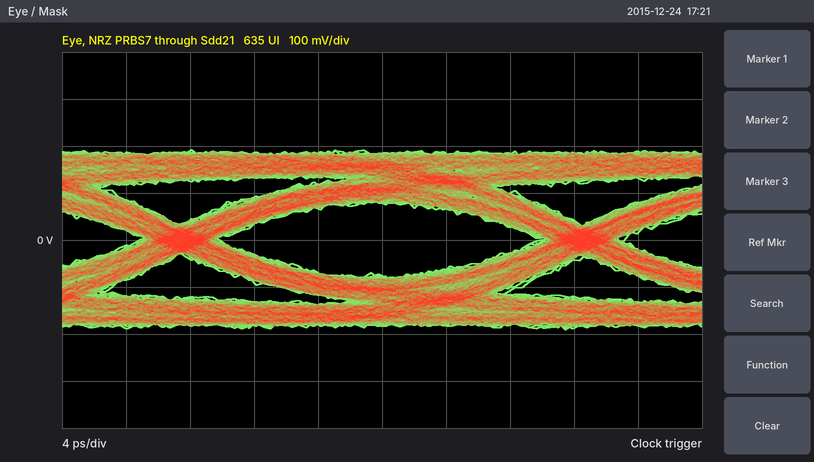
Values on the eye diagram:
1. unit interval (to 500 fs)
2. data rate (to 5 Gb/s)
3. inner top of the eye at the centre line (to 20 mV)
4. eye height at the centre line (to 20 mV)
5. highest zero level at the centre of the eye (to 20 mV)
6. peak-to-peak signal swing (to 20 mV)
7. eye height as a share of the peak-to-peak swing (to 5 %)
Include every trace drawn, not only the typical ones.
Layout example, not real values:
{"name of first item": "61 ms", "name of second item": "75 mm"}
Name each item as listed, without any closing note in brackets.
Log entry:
{"unit interval": "25.0 ps", "data rate": "40 Gb/s", "inner top of the eye at the centre line": "80 mV", "eye height at the centre line": "160 mV", "highest zero level at the centre of the eye": "-80 mV", "peak-to-peak signal swing": "380 mV", "eye height as a share of the peak-to-peak swing": "40 %"}
